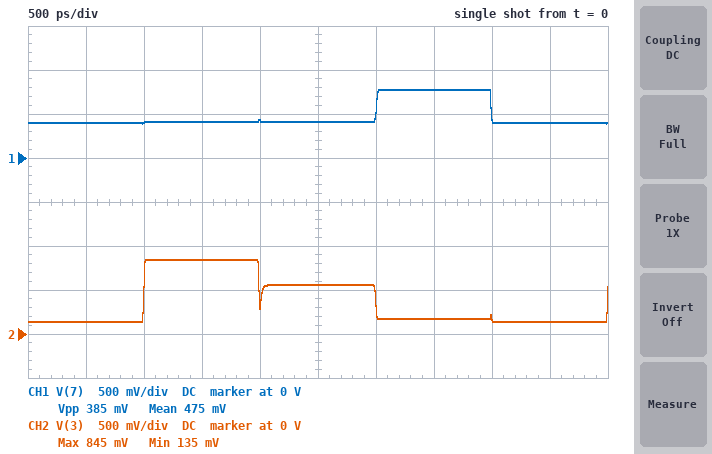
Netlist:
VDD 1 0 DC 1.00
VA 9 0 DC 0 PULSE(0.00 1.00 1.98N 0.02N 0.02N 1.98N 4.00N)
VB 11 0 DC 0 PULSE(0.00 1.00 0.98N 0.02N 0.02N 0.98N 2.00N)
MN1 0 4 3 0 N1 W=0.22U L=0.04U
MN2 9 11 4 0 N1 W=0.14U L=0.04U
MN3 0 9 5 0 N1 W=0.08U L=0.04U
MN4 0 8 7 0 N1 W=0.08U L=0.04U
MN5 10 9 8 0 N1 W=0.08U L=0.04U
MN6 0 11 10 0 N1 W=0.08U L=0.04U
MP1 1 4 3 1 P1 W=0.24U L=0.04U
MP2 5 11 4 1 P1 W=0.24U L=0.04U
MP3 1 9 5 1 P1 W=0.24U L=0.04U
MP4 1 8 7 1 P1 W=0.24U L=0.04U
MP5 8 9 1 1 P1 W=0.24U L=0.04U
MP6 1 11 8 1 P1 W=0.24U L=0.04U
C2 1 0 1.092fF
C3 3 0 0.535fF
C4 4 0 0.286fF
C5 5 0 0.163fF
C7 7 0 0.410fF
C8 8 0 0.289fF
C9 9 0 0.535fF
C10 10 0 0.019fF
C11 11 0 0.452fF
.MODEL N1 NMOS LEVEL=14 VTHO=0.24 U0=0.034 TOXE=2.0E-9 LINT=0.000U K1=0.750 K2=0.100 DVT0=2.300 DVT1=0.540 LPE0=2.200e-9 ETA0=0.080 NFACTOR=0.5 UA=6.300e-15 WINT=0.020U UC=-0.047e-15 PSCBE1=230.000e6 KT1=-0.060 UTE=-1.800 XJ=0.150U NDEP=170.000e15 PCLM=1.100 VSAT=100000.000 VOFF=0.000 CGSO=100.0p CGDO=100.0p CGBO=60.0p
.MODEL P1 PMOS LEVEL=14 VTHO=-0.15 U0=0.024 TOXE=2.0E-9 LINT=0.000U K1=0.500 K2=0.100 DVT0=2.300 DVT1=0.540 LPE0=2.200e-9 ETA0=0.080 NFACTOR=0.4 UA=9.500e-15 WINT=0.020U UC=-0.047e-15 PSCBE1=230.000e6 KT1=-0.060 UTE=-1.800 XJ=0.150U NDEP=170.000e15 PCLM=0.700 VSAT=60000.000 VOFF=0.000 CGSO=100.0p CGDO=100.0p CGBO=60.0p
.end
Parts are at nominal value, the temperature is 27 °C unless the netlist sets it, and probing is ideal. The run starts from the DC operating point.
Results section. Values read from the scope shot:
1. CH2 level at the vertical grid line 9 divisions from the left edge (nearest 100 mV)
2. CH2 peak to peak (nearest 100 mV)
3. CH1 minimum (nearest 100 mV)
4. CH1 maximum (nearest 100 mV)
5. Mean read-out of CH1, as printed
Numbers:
100 mV
700 mV
400 mV
800 mV
475 mV
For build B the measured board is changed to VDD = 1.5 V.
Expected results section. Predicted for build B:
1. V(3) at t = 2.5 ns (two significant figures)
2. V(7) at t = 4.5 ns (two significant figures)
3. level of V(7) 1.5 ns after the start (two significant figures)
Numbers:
300 mV
570 mV
590 mV
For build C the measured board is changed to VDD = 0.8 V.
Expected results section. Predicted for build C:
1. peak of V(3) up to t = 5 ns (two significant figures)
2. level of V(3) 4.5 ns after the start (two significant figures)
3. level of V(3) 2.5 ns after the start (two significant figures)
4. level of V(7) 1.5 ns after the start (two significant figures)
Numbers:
750 mV
110 mV
680 mV
340 mV
